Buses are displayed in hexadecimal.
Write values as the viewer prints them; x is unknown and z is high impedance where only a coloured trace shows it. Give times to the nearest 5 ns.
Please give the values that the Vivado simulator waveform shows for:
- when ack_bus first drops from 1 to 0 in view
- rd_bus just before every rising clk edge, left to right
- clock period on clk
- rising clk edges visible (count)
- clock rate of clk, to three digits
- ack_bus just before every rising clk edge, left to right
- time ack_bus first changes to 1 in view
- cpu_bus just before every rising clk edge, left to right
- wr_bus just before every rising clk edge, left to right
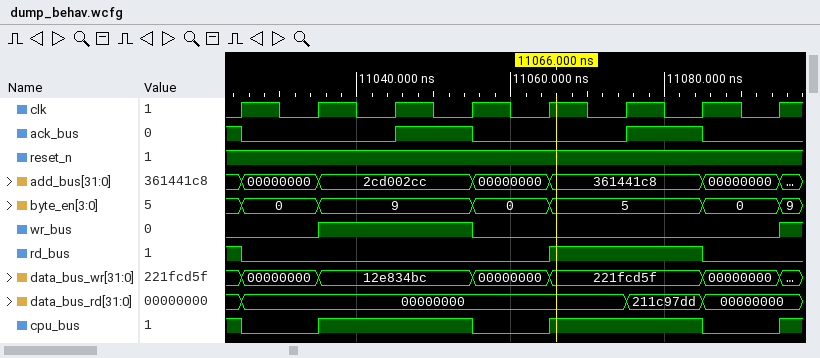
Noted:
11025 ns
1 0 0 0 0 1 1 0
10 ns
8
100 MHz
1 0 0 1 0 0 1 0
11045 ns
1 0 1 1 0 1 1 0
0 0 1 1 0 0 0 0
